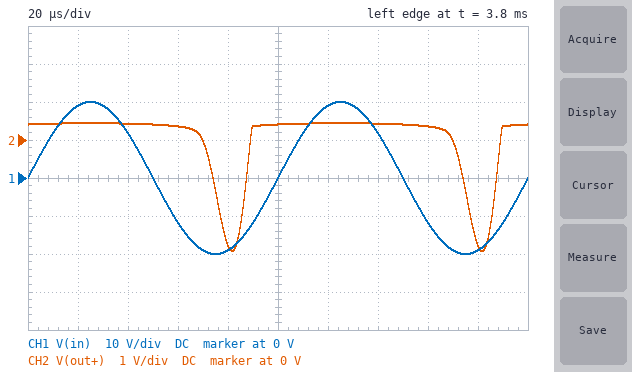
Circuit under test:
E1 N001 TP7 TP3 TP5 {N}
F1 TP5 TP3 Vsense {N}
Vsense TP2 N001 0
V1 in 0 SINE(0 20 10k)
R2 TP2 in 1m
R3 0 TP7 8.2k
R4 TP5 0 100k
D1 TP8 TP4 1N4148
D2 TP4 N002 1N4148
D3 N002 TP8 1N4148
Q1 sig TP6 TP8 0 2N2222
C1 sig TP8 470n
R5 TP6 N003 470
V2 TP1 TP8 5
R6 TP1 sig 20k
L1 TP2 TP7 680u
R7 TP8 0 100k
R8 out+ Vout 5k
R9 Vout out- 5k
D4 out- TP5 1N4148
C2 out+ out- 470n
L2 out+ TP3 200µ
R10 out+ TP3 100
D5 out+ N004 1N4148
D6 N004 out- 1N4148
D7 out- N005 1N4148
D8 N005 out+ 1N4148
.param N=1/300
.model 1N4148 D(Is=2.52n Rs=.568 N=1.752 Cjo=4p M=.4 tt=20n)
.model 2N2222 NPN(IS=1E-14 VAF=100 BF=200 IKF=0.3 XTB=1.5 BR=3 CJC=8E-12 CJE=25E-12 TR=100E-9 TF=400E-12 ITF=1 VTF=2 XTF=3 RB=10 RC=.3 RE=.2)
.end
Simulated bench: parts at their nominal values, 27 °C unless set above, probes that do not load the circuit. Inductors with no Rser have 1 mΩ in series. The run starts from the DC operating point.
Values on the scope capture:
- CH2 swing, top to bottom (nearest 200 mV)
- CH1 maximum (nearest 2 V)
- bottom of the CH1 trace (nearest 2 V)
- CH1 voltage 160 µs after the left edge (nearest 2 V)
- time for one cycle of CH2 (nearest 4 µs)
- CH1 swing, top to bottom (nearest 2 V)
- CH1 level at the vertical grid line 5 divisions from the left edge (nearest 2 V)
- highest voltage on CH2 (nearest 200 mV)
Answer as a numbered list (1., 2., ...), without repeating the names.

1. 3.4 V
2. 20 V
3. -20 V
4. -12 V
5. 100 µs
6. 40 V
7. 0 V
8. 400 mV
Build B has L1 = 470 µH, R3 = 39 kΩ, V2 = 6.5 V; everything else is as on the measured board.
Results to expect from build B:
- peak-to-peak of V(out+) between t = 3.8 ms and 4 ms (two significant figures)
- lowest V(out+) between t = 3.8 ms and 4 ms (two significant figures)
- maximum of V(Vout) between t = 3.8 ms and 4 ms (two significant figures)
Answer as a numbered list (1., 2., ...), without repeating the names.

1. 1.8 V
2. -1.5 V
3. 330 mV
